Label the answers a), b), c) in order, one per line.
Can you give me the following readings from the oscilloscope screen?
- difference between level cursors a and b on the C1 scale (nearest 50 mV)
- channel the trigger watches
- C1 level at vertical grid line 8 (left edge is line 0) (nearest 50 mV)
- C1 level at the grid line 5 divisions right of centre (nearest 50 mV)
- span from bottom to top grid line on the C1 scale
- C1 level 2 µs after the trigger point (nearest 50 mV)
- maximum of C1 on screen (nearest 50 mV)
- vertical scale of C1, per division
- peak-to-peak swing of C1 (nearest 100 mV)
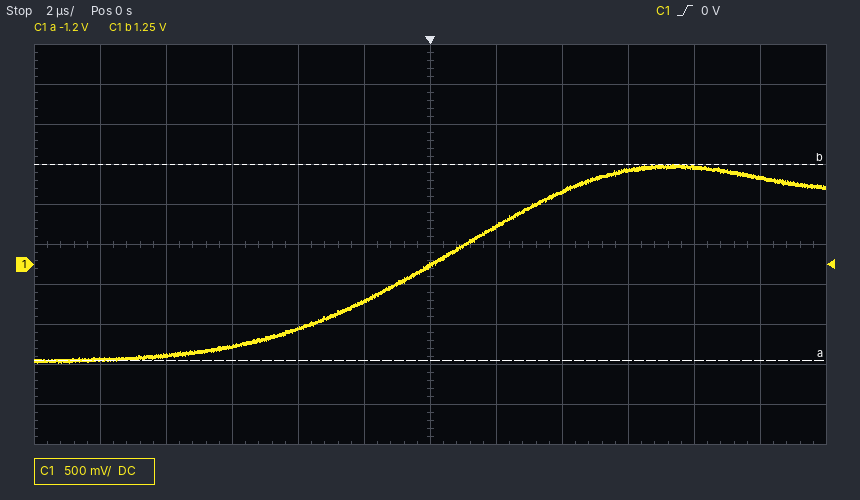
a) 2.45 V
b) C1
c) 900 mV
d) 1.10 V
e) 5 V
f) 500 mV
g) 1.25 V
h) 500 mV
i) 2.50 V
